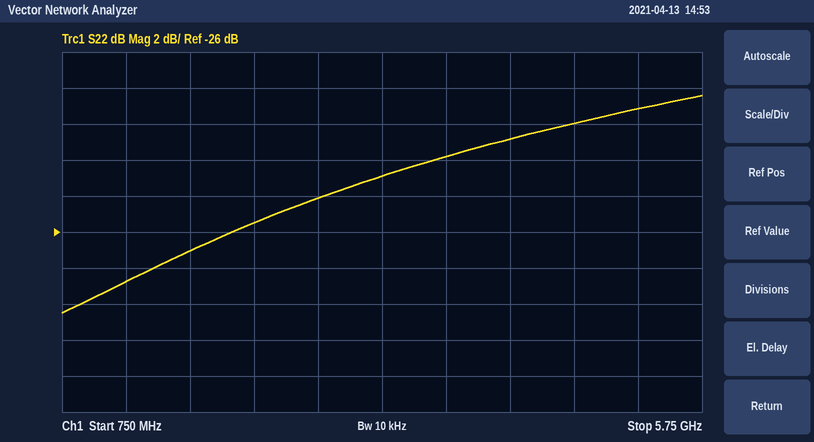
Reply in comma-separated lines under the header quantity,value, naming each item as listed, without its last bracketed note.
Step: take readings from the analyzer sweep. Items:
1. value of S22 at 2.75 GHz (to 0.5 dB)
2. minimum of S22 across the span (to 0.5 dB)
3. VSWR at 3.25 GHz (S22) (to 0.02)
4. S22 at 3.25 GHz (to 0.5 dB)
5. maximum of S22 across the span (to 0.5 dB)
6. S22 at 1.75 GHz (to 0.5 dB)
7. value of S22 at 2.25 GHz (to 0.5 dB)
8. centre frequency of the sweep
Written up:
quantity,value
value of S22 at 2.75 GHz,-24.0 dB
minimum of S22 across the span,-30.5 dB
VSWR at 3.25 GHz (S22),1.16
S22 at 3.25 GHz,-23.0 dB
maximum of S22 across the span,-18.5 dB
S22 at 1.75 GHz,-27.0 dB
value of S22 at 2.25 GHz,-25.5 dB
centre frequency of the sweep,3.25 GHz
